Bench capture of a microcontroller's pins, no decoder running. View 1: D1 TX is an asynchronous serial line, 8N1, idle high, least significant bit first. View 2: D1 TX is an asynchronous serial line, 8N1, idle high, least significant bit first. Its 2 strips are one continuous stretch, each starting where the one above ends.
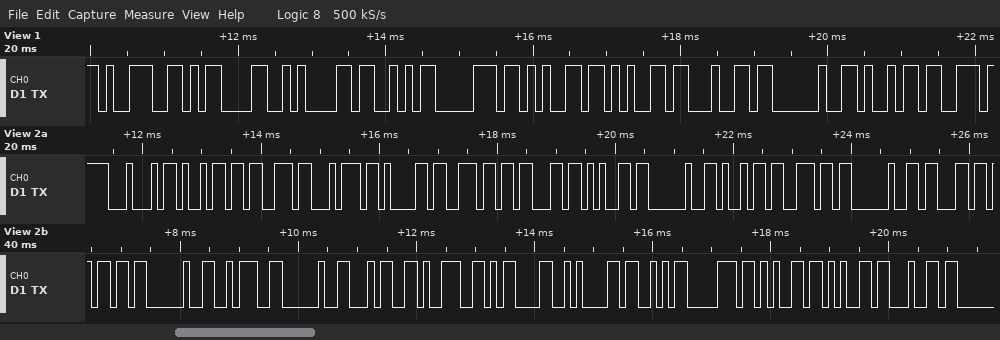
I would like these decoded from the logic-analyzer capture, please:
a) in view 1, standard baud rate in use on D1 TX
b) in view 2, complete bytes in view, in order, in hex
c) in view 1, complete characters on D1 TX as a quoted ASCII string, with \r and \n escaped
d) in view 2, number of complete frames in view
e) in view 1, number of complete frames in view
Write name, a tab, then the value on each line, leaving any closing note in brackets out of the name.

in view 1, standard baud rate in use on D1 TX	9600 baud
in view 2, complete bytes in view, in order, in hex	44 69 73 74 61 6E 63 65 20 69 6E 20 63 6D 20 3A 20 34 39 0D 0A 53 70 65 65 64
in view 1, complete characters on D1 TX as a quoted ASCII string, with \r and \n escaped	"9\r\nSpeed i"
in view 2, number of complete frames in view	26
in view 1, number of complete frames in view	10
